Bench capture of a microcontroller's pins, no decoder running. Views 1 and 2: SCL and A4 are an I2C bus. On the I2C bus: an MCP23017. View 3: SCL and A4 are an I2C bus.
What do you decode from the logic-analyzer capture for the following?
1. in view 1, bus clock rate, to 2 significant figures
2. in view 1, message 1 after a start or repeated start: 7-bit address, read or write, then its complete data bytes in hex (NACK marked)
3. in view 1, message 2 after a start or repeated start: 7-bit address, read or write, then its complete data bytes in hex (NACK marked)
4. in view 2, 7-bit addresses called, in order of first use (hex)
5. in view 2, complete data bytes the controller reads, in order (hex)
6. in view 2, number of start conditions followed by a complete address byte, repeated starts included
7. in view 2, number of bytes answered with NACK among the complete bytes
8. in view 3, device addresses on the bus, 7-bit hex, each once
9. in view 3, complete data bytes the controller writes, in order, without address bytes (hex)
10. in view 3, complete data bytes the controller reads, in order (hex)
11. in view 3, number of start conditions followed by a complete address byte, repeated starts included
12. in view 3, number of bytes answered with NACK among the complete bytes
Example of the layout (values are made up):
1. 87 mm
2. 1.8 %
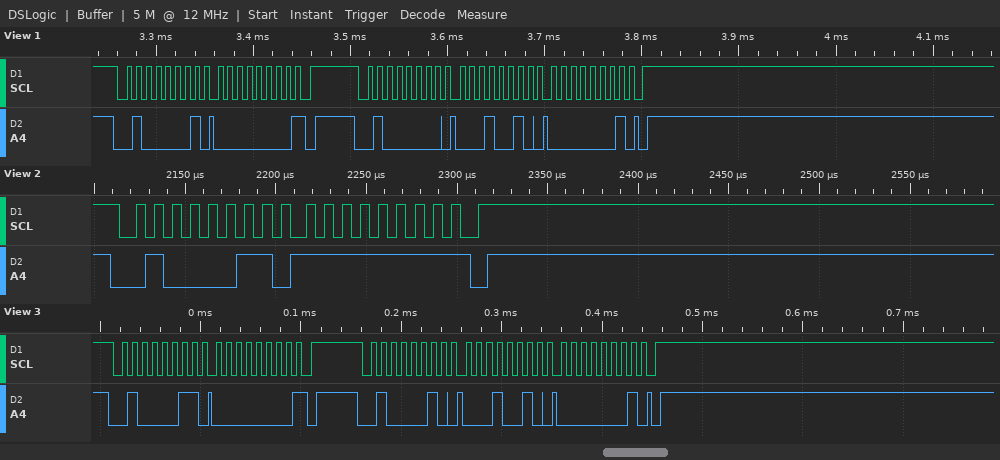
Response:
1. 100 kHz
2. 0x20 read: 00 NACK
3. 0x20 write: 12 01
4. 0x21
5. FF
6. 1
7. 1
8. 0x21
9. 12 01
10. 00
11. 2
12. 1
